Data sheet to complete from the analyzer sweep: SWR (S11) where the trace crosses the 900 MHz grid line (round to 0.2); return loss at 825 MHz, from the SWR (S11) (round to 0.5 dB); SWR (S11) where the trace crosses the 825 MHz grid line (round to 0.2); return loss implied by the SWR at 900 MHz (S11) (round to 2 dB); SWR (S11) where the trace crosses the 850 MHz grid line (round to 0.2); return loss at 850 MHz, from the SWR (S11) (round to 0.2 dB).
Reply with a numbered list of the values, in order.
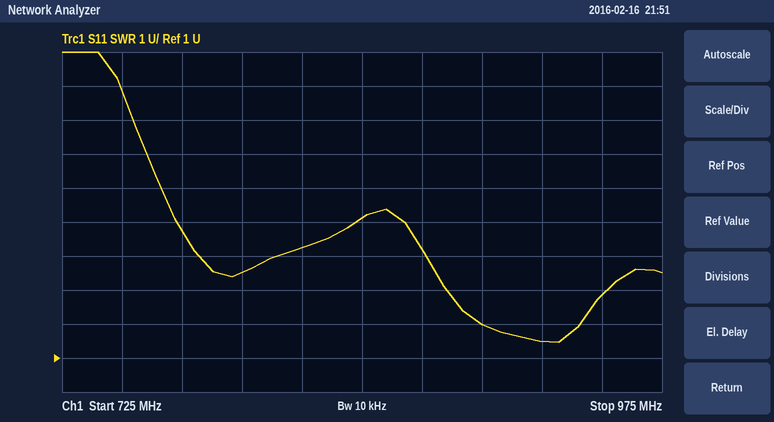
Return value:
1. 2.0
2. 4.0 dB
3. 4.2
4. 10 dB
5. 5.2
6. 3.4 dB
